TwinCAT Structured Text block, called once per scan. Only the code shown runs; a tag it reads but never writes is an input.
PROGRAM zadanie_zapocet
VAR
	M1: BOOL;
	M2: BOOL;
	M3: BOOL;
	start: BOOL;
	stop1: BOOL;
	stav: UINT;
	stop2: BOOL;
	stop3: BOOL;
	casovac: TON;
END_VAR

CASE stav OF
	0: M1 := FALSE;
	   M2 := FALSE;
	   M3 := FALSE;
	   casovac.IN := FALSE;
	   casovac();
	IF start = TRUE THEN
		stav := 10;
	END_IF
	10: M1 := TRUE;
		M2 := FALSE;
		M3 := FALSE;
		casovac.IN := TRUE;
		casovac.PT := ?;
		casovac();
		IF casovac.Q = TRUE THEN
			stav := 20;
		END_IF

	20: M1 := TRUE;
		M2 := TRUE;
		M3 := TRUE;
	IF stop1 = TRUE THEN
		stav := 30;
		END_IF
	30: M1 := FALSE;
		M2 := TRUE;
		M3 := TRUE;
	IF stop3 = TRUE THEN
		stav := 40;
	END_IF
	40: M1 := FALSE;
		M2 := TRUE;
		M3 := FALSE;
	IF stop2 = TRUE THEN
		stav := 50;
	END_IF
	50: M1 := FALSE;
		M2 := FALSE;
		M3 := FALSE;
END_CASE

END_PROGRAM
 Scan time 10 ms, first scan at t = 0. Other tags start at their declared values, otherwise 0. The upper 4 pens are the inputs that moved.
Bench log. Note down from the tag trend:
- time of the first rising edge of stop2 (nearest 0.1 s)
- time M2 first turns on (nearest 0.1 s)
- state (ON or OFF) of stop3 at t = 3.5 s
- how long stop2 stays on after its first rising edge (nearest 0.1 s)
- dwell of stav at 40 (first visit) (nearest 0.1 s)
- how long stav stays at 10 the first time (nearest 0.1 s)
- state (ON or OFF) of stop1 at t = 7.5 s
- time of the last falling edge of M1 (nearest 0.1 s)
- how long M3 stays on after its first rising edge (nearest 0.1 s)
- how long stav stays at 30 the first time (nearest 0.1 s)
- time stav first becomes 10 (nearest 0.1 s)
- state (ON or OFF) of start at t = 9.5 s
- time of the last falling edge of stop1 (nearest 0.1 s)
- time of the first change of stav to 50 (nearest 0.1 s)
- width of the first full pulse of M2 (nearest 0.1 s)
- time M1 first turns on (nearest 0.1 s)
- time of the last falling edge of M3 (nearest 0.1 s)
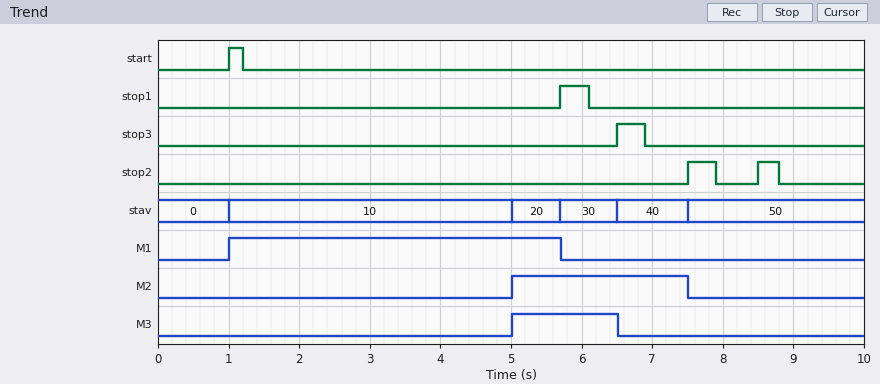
7.5 s
5.0 s
OFF
0.4 s
1.0 s
4.0 s
OFF
5.7 s
1.5 s
0.8 s
1.0 s
OFF
6.1 s
7.5 s
2.5 s
1.0 s
6.5 s
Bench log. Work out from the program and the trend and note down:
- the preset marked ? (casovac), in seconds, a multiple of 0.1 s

4.0 s
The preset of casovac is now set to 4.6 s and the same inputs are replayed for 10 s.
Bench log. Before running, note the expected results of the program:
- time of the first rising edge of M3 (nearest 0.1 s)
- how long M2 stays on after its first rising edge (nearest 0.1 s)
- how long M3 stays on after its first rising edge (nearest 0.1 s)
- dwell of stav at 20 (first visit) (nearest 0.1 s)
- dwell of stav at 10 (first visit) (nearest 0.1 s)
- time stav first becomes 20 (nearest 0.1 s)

5.6 s
1.9 s
0.9 s
0.1 s
4.6 s
5.6 s
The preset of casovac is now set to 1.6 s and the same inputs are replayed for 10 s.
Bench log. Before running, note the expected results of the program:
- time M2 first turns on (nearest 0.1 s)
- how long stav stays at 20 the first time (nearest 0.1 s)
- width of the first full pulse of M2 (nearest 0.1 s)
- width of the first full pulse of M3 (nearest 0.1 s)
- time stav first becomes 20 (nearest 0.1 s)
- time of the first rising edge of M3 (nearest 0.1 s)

2.6 s
3.1 s
4.9 s
3.9 s
2.6 s
2.6 s
